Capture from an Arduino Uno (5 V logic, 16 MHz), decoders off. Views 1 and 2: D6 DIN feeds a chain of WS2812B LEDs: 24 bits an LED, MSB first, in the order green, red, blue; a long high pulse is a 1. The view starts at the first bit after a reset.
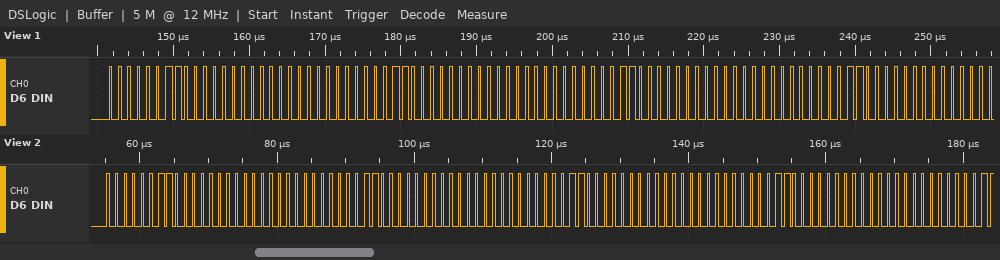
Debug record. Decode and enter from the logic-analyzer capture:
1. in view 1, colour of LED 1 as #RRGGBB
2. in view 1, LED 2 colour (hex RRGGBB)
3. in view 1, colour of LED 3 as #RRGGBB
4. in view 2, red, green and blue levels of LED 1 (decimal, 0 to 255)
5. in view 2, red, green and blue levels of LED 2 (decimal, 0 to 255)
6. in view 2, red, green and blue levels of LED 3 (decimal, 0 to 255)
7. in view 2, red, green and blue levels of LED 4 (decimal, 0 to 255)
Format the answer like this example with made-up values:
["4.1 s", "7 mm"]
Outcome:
["#000300", "#000300", "#000300", "0, 3, 0", "0, 3, 0", "0, 3, 0", "0, 3, 0"]
